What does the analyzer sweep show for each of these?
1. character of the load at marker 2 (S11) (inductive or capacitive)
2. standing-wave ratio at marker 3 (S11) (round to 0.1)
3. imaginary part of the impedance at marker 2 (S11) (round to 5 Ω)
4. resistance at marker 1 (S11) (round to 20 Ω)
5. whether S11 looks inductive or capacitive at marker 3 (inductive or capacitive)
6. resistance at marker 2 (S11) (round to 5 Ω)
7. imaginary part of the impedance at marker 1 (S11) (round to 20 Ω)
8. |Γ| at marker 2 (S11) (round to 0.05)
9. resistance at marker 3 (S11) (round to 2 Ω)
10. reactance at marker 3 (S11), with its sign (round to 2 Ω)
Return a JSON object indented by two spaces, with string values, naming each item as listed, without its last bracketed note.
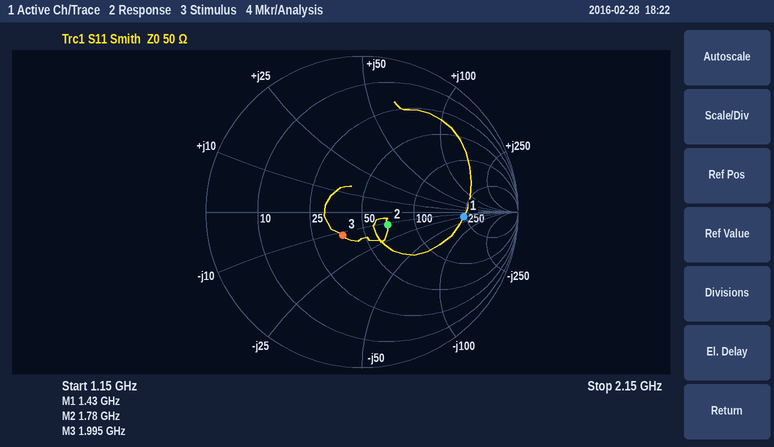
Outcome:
{
  "character of the load at marker 2 (S11)": "capacitive",
  "standing-wave ratio at marker 3 (S11)": "1.5",
  "imaginary part of the impedance at marker 2 (S11)": "-10 Ω",
  "resistance at marker 1 (S11)": "240 Ω",
  "whether S11 looks inductive or capacitive at marker 3": "capacitive",
  "resistance at marker 2 (S11)": "70 Ω",
  "imaginary part of the impedance at marker 1 (S11)": "-20 Ω",
  "|Γ| at marker 2 (S11)": "0.20",
  "resistance at marker 3 (S11)": "38 Ω",
  "reactance at marker 3 (S11), with its sign": "-12 Ω"
}
